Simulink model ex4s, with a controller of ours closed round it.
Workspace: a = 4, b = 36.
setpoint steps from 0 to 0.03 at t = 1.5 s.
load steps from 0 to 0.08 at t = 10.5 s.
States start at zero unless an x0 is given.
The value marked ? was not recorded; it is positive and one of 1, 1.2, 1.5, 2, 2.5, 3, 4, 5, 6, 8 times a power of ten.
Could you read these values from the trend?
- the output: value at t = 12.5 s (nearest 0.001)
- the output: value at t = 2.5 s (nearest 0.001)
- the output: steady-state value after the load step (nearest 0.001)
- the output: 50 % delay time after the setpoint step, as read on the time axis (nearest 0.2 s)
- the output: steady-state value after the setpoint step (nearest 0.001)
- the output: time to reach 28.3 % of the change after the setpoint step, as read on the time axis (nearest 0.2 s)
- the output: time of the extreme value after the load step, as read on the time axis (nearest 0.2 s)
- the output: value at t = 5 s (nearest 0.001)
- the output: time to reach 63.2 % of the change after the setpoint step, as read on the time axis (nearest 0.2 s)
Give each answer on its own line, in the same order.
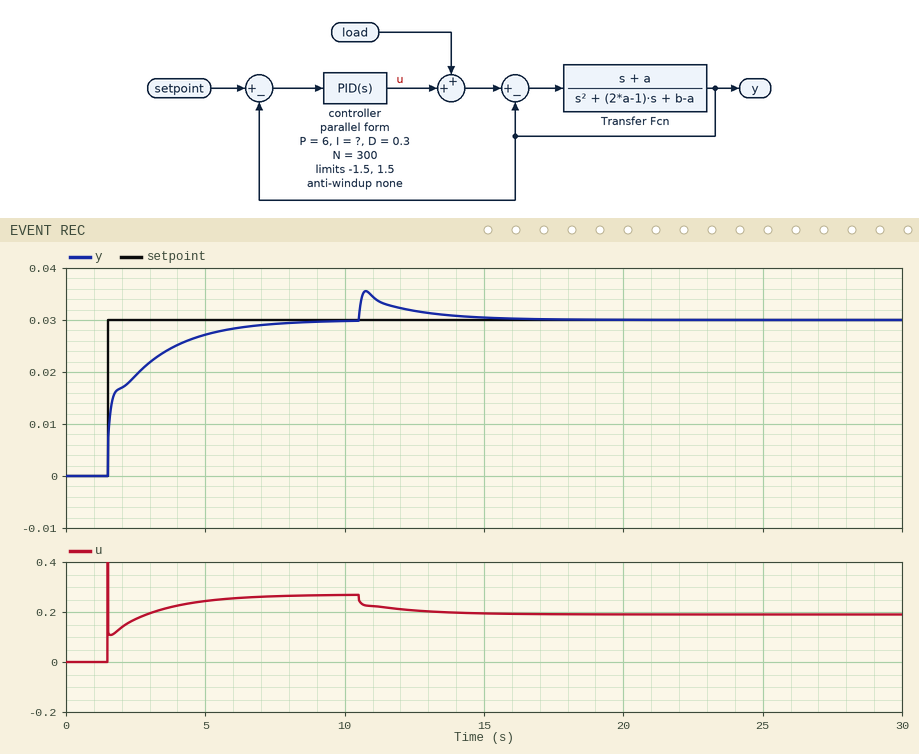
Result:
0.032
0.019
0.030
1.6 s
0.030
1.6 s
10.8 s
0.027
2.4 s
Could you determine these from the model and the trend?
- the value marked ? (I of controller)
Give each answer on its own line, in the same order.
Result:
8
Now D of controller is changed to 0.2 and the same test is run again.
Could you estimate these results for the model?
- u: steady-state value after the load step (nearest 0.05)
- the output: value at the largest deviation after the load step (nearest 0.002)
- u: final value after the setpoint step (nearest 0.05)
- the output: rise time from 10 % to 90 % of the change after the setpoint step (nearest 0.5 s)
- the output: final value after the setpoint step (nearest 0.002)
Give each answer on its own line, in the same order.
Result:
0.20
0.036
0.25
3.5 s
0.030
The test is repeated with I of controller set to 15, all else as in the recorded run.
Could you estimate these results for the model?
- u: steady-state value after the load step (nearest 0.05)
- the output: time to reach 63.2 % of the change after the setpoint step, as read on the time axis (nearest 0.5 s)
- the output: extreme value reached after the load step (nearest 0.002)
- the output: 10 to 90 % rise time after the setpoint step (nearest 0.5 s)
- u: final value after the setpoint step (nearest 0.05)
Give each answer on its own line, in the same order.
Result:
0.20
2.0 s
0.036
2.0 s
0.25
